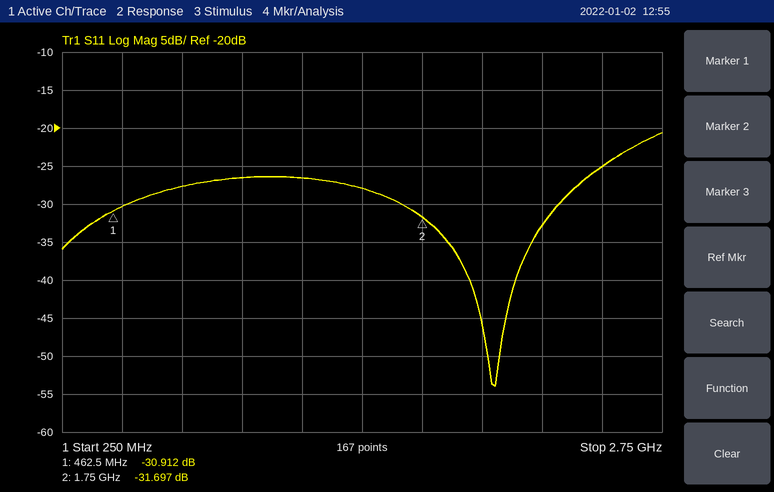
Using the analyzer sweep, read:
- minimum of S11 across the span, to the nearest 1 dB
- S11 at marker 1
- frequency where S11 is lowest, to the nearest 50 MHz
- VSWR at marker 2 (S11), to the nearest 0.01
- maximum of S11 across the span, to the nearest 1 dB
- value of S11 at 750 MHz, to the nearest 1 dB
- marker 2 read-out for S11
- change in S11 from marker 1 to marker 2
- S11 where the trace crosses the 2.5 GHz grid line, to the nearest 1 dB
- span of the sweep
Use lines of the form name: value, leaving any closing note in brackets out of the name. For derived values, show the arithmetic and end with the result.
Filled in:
minimum of S11 across the span, to the nearest 1 dB: -54 dB
S11 at marker 1: -30.912 dB
frequency where S11 is lowest, to the nearest 50 MHz: 2.05 GHz
VSWR at marker 2 (S11), to the nearest 0.01: (1 + 0.0260)/(1 − 0.0260) ≈ 1.05
maximum of S11 across the span, to the nearest 1 dB: -21 dB
value of S11 at 750 MHz, to the nearest 1 dB: -28 dB
marker 2 read-out for S11: -31.697 dB
change in S11 from marker 1 to marker 2: -31.697 − (-30.912) = -0.785 dB
S11 where the trace crosses the 2.5 GHz grid line, to the nearest 1 dB: -25 dB
span of the sweep: 2.5 GHz
